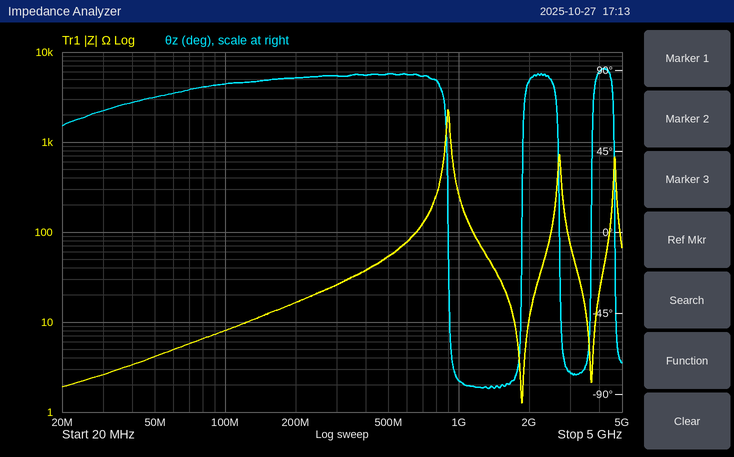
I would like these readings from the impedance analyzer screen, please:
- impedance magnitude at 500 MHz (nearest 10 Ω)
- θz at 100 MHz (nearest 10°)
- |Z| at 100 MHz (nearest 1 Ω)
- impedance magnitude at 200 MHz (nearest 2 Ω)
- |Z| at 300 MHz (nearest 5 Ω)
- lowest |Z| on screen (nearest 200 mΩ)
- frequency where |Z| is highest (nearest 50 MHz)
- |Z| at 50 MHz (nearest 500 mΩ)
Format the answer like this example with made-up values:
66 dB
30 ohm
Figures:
50 Ω
80°
8 Ω
16 Ω
25 Ω
1.2 Ω
900 MHz
4.0 Ω
